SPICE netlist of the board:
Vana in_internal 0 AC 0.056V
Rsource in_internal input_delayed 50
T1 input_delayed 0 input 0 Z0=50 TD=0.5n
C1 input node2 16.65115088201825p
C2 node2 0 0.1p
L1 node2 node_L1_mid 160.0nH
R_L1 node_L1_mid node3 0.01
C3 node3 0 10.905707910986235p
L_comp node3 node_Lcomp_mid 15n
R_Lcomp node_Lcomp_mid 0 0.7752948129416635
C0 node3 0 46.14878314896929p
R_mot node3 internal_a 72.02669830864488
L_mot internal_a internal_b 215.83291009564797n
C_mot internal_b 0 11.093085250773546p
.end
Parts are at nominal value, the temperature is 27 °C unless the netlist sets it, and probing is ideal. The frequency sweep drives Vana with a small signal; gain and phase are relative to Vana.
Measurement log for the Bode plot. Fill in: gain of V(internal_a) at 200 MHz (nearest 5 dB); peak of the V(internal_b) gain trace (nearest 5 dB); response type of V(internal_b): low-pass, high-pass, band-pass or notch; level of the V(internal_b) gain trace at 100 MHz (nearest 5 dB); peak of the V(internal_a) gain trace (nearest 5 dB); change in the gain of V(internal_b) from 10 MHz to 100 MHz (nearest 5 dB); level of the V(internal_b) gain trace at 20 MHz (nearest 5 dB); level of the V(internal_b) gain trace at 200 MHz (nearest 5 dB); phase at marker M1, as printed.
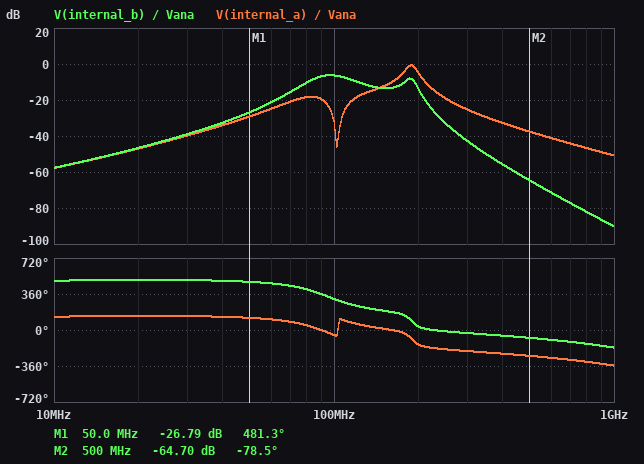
-5 dB
-5 dB
band-pass
-5 dB
0 dB
50 dB
-45 dB
-15 dB
481.3 deg
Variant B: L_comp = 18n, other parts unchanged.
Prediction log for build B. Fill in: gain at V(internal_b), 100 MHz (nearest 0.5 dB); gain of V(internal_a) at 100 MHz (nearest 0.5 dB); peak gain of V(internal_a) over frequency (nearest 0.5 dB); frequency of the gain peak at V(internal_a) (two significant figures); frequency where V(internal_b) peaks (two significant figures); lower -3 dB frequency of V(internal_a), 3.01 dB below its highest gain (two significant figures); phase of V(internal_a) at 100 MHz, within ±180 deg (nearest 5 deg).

-4.5 dB
-29.5 dB
-0.5 dB
180 MHz
96 MHz
170 MHz
-55 deg
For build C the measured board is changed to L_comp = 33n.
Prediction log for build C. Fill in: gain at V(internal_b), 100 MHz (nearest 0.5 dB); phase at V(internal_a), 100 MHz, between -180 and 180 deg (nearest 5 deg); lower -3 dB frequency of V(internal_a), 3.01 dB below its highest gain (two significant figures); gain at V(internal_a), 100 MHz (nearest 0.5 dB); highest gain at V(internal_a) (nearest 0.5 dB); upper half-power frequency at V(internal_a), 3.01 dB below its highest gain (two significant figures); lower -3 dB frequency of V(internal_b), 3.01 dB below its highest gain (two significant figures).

0.5 dB
-90 deg
130 MHz
-25.0 dB
-3.0 dB
160 MHz
74 MHz
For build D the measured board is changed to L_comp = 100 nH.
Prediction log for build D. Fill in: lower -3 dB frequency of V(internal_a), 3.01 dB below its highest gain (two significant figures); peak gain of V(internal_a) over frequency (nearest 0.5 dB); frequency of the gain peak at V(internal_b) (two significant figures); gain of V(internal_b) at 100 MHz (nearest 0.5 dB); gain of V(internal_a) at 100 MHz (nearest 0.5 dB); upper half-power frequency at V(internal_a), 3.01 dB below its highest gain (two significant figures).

49 MHz
3.0 dB
53 MHz
0 dB
-25.0 dB
57 MHz
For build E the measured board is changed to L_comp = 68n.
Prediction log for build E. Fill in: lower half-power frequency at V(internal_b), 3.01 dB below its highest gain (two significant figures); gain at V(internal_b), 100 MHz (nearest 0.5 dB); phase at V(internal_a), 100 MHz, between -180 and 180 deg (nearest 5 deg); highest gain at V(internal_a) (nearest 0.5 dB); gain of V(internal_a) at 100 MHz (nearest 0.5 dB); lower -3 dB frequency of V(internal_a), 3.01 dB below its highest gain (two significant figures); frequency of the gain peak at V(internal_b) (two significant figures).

58 MHz
1.0 dB
-125 deg
0 dB
-24.5 dB
57 MHz
63 MHz
